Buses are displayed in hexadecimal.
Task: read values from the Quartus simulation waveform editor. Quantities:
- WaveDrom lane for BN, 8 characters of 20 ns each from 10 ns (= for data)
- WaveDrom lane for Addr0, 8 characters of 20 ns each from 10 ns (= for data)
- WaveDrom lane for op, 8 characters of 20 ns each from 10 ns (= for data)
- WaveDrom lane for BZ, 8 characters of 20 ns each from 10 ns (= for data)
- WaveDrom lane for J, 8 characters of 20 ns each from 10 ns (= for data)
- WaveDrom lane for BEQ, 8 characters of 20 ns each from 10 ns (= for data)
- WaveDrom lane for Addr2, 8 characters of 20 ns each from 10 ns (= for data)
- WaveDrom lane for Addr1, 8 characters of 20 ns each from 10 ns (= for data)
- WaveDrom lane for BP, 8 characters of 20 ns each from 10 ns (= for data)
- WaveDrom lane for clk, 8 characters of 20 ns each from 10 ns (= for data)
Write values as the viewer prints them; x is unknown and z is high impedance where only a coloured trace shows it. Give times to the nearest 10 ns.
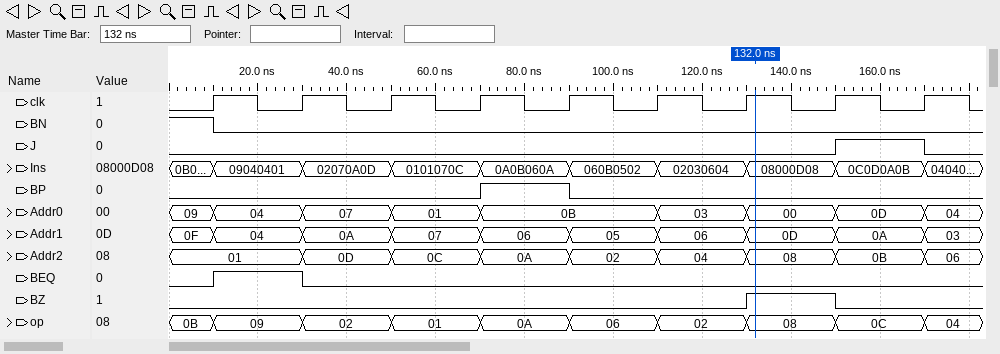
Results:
{name: 'BN', wave: '0.......'}
{name: 'Addr0', wave: '====.===', data: '04 07 01 0B 03 00 0D'}
{name: 'op', wave: '========', data: '09 02 01 0A 06 02 08 0C'}
{name: 'BZ', wave: '0.....10'}
{name: 'J', wave: '0......1'}
{name: 'BEQ', wave: '10......'}
{name: 'Addr2', wave: '========', data: '01 0D 0C 0A 02 04 08 0B'}
{name: 'Addr1', wave: '========', data: '04 0A 07 06 05 06 0D 0A'}
{name: 'BP', wave: '0..10...'}
{name: 'clk', wave: 'p.......'}
